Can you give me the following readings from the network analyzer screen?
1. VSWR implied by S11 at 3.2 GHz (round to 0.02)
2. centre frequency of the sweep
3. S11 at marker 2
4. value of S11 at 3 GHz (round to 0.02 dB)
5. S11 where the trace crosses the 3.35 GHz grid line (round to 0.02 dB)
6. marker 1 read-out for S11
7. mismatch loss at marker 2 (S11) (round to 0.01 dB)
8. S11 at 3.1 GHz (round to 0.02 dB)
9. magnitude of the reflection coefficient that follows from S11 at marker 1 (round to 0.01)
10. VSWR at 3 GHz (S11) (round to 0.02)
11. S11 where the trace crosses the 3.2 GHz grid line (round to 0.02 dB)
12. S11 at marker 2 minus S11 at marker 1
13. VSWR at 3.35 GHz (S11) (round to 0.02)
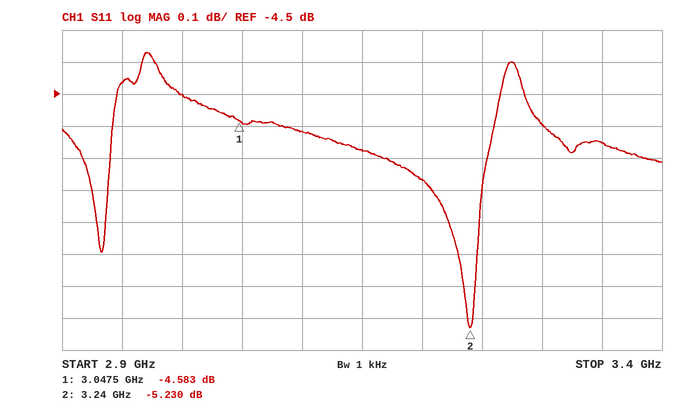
3.74
3.15 GHz
-5.230 dB
-4.50 dB
-4.66 dB
-4.583 dB
1.55 dB
-4.62 dB
0.59
3.94
-4.76 dB
-0.647 dB
3.82
